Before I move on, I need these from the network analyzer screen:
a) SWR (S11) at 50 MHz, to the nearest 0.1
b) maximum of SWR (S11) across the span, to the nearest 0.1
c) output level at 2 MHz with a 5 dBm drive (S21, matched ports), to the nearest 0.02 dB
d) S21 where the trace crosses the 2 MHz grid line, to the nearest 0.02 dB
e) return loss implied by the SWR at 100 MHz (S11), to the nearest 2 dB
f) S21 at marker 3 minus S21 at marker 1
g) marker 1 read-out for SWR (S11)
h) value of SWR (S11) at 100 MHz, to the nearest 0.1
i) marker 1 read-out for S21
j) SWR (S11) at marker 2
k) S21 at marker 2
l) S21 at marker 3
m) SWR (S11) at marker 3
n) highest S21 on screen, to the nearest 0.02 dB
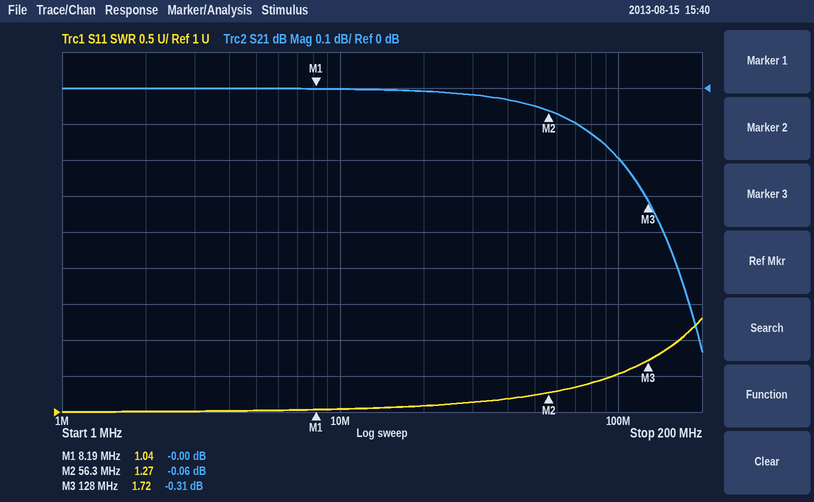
1.2
2.3
5.00 dBm
0.00 dB
14 dB
-0.31 dB
1.04
1.5
-0.00 dB
1.27
-0.06 dB
-0.31 dB
1.72
0.00 dB
